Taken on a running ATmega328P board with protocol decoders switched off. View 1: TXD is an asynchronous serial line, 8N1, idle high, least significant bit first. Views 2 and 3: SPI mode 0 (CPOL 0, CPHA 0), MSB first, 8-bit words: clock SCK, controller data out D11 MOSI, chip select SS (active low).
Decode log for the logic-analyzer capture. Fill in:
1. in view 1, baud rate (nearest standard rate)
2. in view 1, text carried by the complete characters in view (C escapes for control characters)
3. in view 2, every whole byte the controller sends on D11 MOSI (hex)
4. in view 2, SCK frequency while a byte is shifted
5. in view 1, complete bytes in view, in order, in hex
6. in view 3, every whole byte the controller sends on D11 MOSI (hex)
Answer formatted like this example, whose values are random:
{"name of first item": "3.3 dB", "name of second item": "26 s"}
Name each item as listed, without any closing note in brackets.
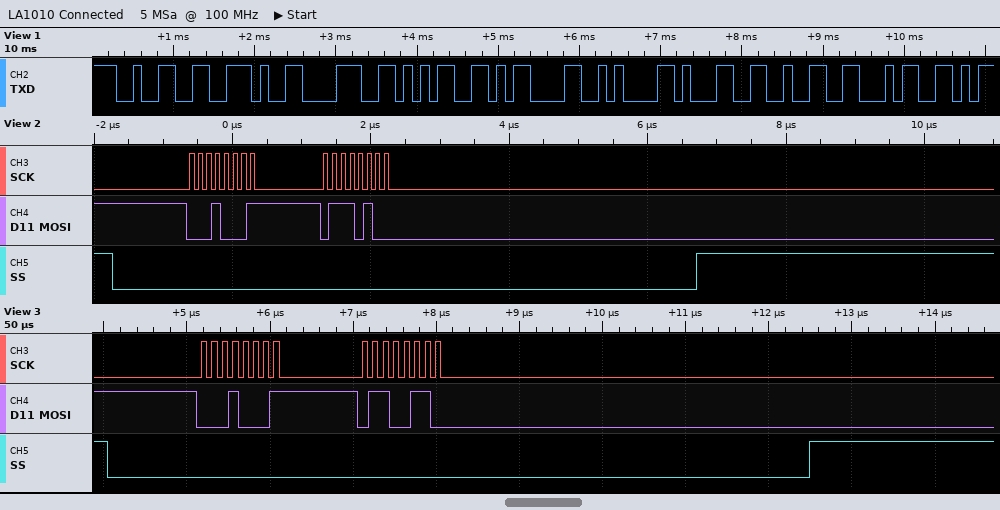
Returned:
{"in view 1, baud rate": "9600 baud", "in view 1, text carried by the complete characters in view": "\"2.85\\r\\n124\"", "in view 2, every whole byte the controller sends on D11 MOSI": "0x11 0x74", "in view 2, SCK frequency while a byte is shifted": "8 MHz", "in view 1, complete bytes in view, in order, in hex": "32 2E 38 35 0D 0A 31 32 34", "in view 3, every whole byte the controller sends on D11 MOSI": "11 66"}
